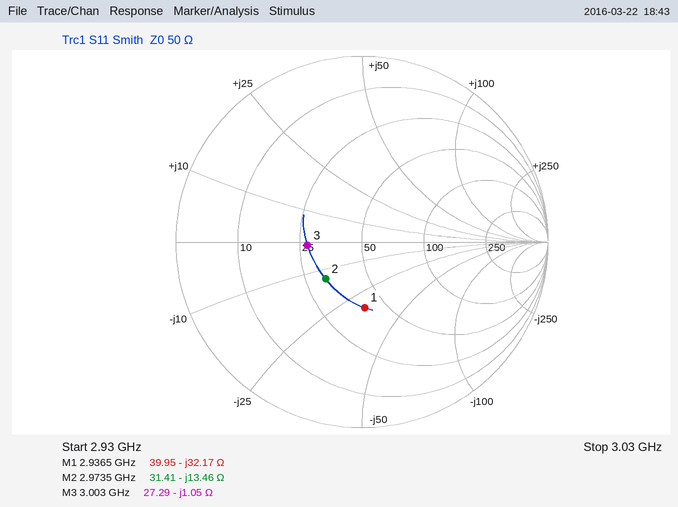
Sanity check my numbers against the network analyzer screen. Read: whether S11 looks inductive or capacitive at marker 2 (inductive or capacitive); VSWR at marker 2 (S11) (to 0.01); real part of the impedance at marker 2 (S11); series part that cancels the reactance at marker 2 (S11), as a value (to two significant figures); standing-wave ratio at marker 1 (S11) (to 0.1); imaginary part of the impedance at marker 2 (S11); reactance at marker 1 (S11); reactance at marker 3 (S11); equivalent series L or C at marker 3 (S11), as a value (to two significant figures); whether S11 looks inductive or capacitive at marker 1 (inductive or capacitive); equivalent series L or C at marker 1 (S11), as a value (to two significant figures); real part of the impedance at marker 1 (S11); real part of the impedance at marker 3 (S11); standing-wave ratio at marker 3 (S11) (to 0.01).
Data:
capacitive
1.77
31.41 Ω
720 pH
2.1
-13.46 Ω
-32.17 Ω
-1.05 Ω
50 pF
capacitive
1.7 pF
39.95 Ω
27.29 Ω
1.83
